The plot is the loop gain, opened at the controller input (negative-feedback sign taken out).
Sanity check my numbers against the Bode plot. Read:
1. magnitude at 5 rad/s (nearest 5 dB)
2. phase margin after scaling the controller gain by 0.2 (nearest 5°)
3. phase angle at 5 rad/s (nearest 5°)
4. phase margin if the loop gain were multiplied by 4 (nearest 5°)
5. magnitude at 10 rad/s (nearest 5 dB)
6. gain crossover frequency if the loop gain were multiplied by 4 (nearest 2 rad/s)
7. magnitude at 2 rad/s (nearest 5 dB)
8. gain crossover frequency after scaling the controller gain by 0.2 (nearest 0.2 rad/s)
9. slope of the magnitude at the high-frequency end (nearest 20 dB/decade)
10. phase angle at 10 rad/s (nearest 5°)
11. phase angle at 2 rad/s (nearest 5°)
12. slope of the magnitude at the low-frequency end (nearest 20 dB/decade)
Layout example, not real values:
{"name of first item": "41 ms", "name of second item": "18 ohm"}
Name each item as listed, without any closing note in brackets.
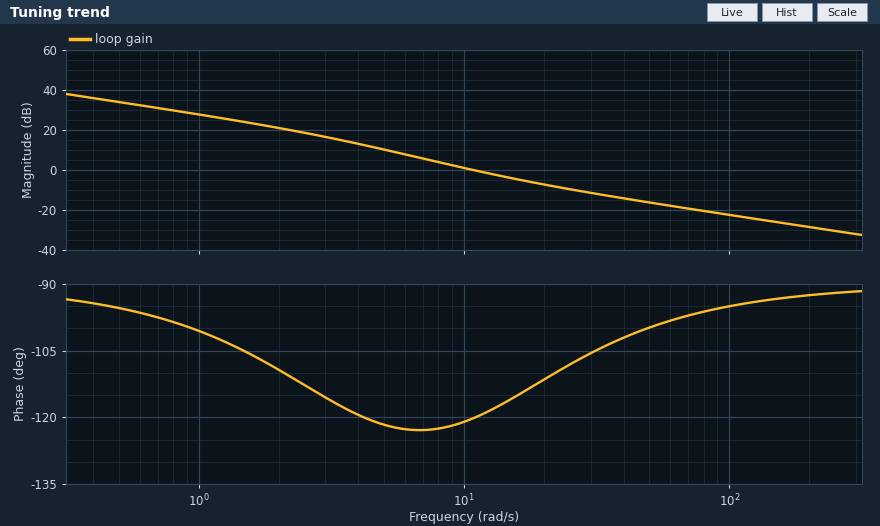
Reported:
{"magnitude at 5 rad/s": "10 dB", "phase margin after scaling the controller gain by 0.2": "60°", "phase angle at 5 rad/s": "-120°", "phase margin if the loop gain were multiplied by 4": "75°", "magnitude at 10 rad/s": "0 dB", "gain crossover frequency if the loop gain were multiplied by 4": "32 rad/s", "magnitude at 2 rad/s": "20 dB", "gain crossover frequency after scaling the controller gain by 0.2": "3.8 rad/s", "slope of the magnitude at the high-frequency end": "-20 dB/decade", "phase angle at 10 rad/s": "-120°", "phase angle at 2 rad/s": "-110°", "slope of the magnitude at the low-frequency end": "-20 dB/decade"}
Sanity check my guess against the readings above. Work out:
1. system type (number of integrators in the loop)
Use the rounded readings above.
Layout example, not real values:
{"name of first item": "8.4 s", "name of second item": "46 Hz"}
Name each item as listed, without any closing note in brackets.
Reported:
{"system type": "1"}
